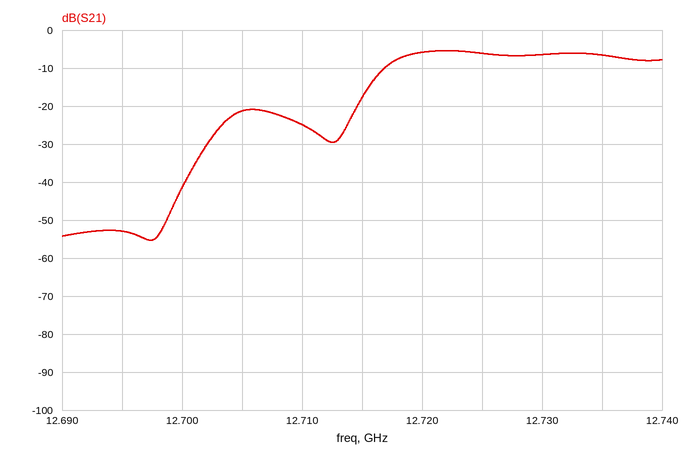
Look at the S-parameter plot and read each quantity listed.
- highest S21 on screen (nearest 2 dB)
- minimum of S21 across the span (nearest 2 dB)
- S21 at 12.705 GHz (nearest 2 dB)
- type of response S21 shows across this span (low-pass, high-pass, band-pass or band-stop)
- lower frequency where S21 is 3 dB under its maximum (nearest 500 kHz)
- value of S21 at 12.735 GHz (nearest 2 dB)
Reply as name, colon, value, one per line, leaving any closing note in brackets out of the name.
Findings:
highest S21 on screen: -6 dB
minimum of S21 across the span: -56 dB
S21 at 12.705 GHz: -22 dB
type of response S21 shows across this span: high-pass
lower frequency where S21 is 3 dB under its maximum: 12.7175 GHz
value of S21 at 12.735 GHz: -6 dB
